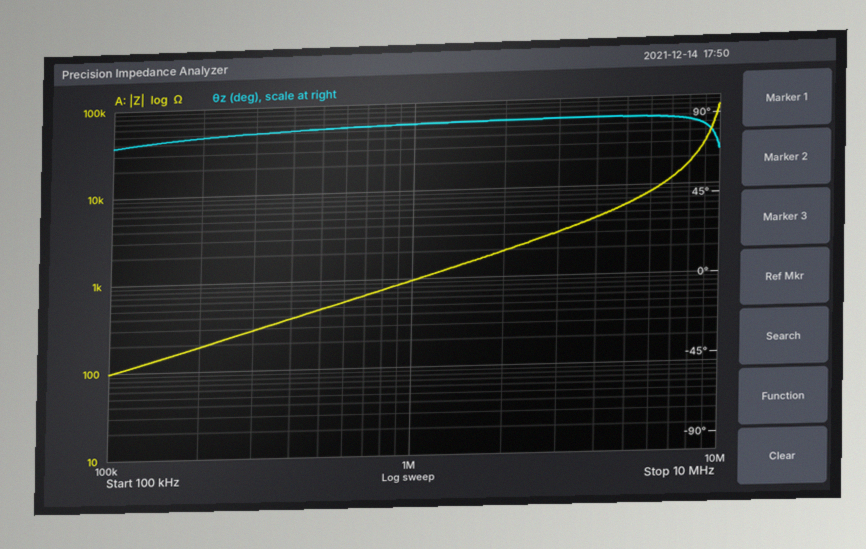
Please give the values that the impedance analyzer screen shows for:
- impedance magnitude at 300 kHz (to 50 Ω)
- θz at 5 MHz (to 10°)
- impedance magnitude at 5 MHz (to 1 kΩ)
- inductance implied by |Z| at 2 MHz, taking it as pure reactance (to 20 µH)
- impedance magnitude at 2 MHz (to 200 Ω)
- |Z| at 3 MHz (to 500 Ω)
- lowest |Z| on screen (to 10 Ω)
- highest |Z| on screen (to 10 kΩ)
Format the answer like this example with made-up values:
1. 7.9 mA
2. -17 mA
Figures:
1. 300 Ω
2. 90°
3. 6 kΩ
4. 160 µH
5. 2.0 kΩ
6. 3.0 kΩ
7. 100 Ω
8. 80 kΩ
